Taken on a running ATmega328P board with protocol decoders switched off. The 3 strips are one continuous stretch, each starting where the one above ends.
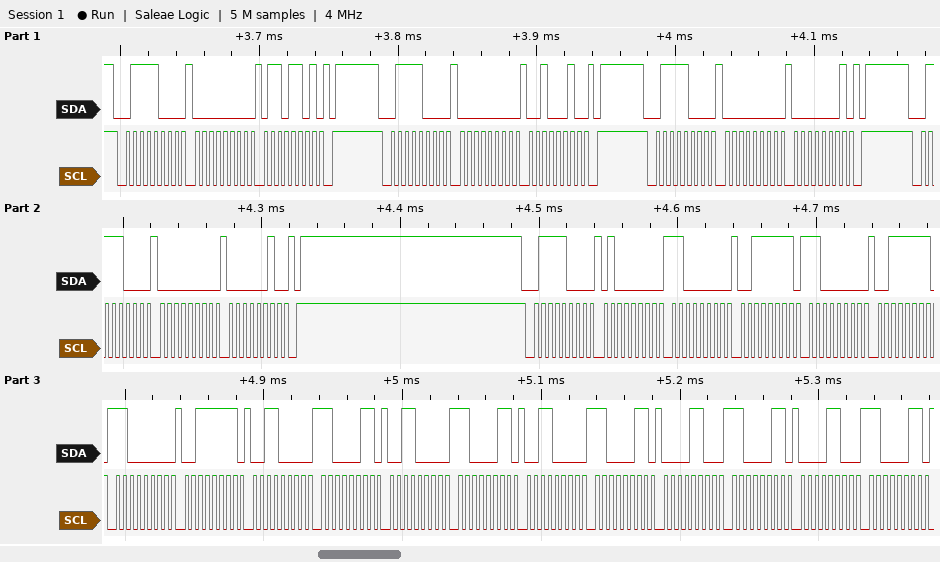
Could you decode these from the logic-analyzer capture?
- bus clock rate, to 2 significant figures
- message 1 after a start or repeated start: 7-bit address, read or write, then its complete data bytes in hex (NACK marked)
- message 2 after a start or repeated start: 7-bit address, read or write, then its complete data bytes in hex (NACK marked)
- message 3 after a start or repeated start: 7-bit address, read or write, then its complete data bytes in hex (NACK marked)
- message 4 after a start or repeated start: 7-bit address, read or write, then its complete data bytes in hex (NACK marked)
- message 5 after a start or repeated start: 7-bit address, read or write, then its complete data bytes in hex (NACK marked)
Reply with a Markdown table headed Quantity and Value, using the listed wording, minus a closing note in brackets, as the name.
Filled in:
| Quantity | Value |
|---|---|
| bus clock rate, to 2 significant figures | 200 kHz |
| message 1 after a start or repeated start: 7-bit address, read or write, then its complete data bytes in hex | 0x3C write: 00 6D |
| message 2 after a start or repeated start: 7-bit address, read or write, then its complete data bytes in hex | 0x3C write: 00 22 |
| message 3 after a start or repeated start: 7-bit address, read or write, then its complete data bytes in hex | 0x3C write: 00 01 |
| message 4 after a start or repeated start: 7-bit address, read or write, then its complete data bytes in hex | 0x3C write: 00 02 |
| message 5 after a start or repeated start: 7-bit address, read or write, then its complete data bytes in hex | 0x3C write: 40 C0 3F C0 3F C0 3F 30 C3 30 C3 30 C3 0C C3 0C C3 |
